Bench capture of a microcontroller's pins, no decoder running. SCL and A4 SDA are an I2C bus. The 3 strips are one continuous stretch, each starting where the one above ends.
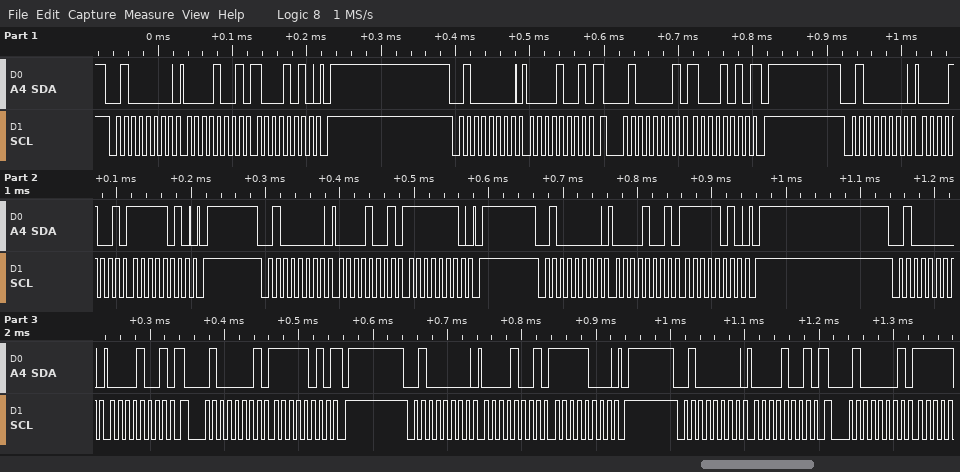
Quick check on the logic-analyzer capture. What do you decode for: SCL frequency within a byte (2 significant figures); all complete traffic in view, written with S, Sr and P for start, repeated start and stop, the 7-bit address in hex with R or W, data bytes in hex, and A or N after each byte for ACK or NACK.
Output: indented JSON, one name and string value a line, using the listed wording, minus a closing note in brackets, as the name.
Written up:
{
  "SCL frequency within a byte": "100 kHz",
  "all complete traffic in view, written with S, Sr and P for start, repeated start and stop, the 7-bit address in hex with R or W, data bytes in hex, and A or N after each byte for ACK or NACK": "S 20W A 09 A 8A A P S 20W A 09 A Sr 20R A 8A N P S 20W A 09 A FA A P S 20W A 09 A FE A P S 20W A 09 A FA A P S 20W A 09 A Sr 20R A FA N P S 20W A 09 A F8 A P S 20W A 09 A Sr 20R A"
}
